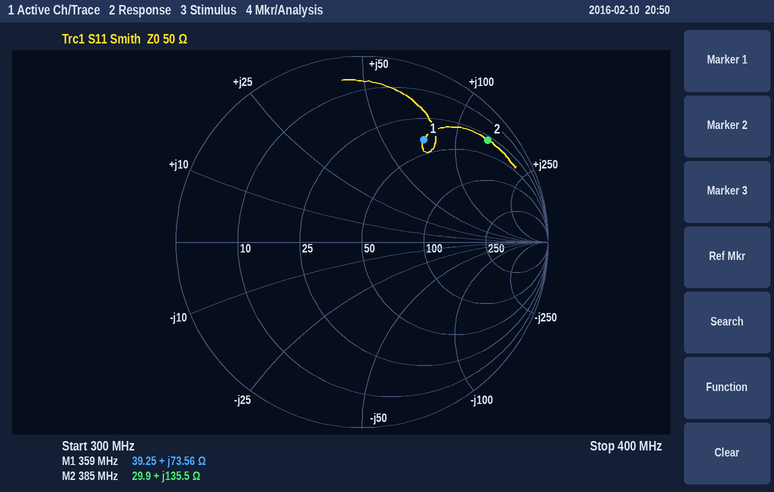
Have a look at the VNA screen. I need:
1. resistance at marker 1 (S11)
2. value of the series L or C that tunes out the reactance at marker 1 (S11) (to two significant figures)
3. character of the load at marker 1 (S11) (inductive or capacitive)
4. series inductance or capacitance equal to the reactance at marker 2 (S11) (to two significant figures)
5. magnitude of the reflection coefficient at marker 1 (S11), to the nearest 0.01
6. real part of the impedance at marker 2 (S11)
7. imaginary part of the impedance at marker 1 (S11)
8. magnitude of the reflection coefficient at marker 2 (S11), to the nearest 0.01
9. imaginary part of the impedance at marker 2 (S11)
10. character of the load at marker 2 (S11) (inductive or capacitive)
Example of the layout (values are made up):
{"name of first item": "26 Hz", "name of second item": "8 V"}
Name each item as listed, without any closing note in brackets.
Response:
{"resistance at marker 1": "39.25 Ω", "value of the series L or C that tunes out the reactance at marker 1 (S11)": "6.0 pF", "character of the load at marker 1 (S11)": "inductive", "series inductance or capacitance equal to the reactance at marker 2 (S11)": "56 nH", "magnitude of the reflection coefficient at marker 1 (S11), to the nearest 0.01": "0.64", "real part of the impedance at marker 2": "29.9 Ω", "imaginary part of the impedance at marker 1": "+73.56 Ω", "magnitude of the reflection coefficient at marker 2 (S11), to the nearest 0.01": "0.87", "imaginary part of the impedance at marker 2": "+135.5 Ω", "character of the load at marker 2 (S11)": "inductive"}
